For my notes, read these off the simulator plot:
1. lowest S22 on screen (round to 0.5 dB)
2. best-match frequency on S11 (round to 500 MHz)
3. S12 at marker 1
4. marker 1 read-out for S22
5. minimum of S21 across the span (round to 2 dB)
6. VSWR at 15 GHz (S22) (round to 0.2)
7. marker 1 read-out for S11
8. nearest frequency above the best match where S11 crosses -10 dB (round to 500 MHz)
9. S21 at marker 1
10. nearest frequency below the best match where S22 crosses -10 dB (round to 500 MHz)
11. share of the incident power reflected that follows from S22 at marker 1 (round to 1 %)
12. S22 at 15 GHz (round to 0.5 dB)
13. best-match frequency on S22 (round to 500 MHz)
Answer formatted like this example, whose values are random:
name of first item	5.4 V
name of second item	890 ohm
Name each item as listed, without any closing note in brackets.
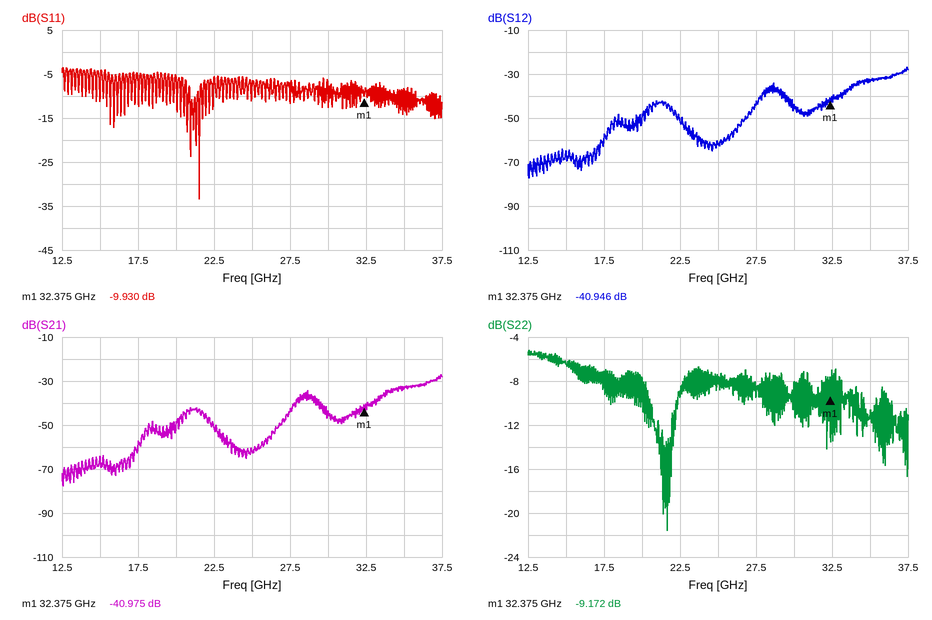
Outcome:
lowest S22 on screen	-21.5 dB
best-match frequency on S11	21.5 GHz
S12 at marker 1	-40.946 dB
marker 1 read-out for S22	-9.172 dB
minimum of S21 across the span	-78 dB
VSWR at 15 GHz (S22)	2.8
marker 1 read-out for S11	-9.930 dB
nearest frequency above the best match where S11 crosses -10 dB	21.5 GHz
S21 at marker 1	-40.975 dB
nearest frequency below the best match where S22 crosses -10 dB	20.5 GHz
share of the incident power reflected that follows from S22 at marker 1	12 %
S22 at 15 GHz	-6.5 dB
best-match frequency on S22	21.5 GHz
